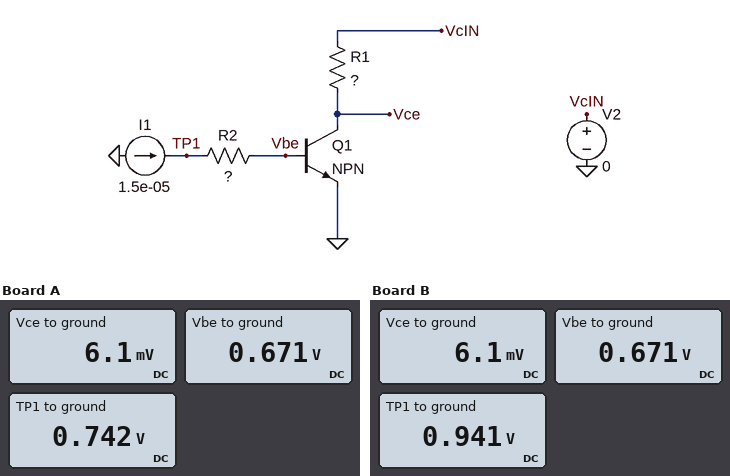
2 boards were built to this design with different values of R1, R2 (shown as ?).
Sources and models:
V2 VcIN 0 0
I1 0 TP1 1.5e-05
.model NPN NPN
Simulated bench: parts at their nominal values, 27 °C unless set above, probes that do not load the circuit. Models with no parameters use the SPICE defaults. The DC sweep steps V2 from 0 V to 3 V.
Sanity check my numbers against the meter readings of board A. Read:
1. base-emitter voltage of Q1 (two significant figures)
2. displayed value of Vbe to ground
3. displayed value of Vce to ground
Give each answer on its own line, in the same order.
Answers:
670 mV
0.671 V
6.1 mV
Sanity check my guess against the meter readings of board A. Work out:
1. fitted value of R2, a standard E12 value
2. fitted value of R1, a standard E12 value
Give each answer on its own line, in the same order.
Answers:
4.7 kΩ
560 Ω
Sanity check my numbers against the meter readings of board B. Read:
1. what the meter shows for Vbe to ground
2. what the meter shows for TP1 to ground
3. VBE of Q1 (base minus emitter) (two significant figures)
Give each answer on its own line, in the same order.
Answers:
0.671 V
0.941 V
670 mV
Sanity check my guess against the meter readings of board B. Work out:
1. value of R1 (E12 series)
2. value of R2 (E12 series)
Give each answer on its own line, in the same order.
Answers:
560 Ω
18 kΩ
